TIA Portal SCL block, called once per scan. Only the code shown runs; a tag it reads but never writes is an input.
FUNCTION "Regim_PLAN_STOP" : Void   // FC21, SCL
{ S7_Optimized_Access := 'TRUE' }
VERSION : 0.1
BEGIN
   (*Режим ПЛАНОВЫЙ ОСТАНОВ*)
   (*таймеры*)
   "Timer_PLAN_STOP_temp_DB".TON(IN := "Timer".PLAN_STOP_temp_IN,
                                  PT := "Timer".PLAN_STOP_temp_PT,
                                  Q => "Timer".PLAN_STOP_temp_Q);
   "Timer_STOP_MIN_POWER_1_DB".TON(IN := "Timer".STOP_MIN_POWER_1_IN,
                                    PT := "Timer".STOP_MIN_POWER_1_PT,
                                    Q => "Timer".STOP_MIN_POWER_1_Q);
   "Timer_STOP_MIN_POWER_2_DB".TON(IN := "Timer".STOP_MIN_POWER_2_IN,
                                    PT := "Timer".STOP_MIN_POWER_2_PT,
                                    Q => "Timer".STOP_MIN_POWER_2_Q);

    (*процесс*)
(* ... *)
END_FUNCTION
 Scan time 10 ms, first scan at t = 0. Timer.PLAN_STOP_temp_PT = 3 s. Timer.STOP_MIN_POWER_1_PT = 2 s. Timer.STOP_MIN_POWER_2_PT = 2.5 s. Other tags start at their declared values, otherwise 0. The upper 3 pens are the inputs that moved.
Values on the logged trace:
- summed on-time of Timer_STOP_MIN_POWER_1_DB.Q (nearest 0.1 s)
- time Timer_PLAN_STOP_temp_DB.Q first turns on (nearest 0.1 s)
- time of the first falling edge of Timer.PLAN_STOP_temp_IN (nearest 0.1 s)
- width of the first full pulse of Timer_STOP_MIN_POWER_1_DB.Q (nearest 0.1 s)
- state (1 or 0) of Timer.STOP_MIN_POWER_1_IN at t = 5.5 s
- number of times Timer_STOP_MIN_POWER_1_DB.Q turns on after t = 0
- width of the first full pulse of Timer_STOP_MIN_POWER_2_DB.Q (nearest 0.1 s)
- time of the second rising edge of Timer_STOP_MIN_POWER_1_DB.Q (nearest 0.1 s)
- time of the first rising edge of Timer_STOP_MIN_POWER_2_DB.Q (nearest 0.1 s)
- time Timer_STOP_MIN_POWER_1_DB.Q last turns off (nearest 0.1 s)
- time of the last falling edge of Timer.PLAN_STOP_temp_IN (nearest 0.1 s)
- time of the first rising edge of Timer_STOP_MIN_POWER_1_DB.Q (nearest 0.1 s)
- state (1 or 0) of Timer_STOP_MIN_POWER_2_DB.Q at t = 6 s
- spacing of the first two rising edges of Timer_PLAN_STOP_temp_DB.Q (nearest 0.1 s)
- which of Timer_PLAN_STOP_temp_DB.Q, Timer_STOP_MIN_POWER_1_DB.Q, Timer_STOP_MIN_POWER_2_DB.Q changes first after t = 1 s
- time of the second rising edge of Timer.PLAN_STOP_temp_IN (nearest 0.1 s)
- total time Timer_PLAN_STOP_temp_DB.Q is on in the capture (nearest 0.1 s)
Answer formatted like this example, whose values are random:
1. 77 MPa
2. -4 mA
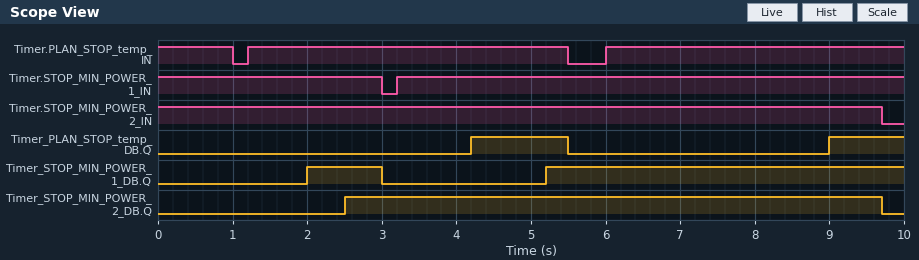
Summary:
1. 5.8 s
2. 4.2 s
3. 1.0 s
4. 1.0 s
5. 1
6. 2
7. 7.2 s
8. 5.2 s
9. 2.5 s
10. 3.0 s
11. 5.5 s
12. 2.0 s
13. 1
14. 4.8 s
15. Timer_STOP_MIN_POWER_1_DB.Q
16. 6.0 s
17. 2.3 s
